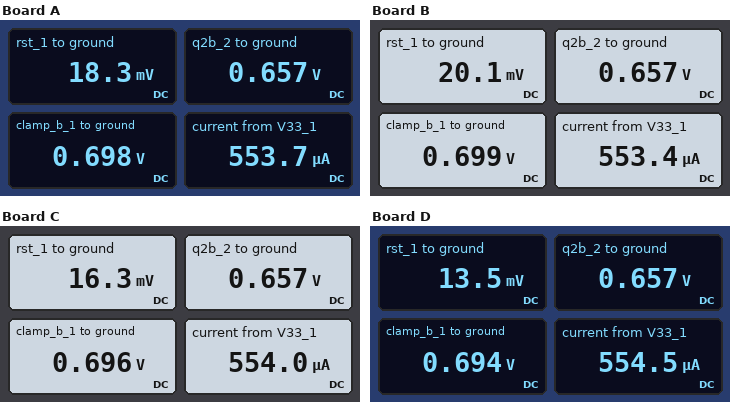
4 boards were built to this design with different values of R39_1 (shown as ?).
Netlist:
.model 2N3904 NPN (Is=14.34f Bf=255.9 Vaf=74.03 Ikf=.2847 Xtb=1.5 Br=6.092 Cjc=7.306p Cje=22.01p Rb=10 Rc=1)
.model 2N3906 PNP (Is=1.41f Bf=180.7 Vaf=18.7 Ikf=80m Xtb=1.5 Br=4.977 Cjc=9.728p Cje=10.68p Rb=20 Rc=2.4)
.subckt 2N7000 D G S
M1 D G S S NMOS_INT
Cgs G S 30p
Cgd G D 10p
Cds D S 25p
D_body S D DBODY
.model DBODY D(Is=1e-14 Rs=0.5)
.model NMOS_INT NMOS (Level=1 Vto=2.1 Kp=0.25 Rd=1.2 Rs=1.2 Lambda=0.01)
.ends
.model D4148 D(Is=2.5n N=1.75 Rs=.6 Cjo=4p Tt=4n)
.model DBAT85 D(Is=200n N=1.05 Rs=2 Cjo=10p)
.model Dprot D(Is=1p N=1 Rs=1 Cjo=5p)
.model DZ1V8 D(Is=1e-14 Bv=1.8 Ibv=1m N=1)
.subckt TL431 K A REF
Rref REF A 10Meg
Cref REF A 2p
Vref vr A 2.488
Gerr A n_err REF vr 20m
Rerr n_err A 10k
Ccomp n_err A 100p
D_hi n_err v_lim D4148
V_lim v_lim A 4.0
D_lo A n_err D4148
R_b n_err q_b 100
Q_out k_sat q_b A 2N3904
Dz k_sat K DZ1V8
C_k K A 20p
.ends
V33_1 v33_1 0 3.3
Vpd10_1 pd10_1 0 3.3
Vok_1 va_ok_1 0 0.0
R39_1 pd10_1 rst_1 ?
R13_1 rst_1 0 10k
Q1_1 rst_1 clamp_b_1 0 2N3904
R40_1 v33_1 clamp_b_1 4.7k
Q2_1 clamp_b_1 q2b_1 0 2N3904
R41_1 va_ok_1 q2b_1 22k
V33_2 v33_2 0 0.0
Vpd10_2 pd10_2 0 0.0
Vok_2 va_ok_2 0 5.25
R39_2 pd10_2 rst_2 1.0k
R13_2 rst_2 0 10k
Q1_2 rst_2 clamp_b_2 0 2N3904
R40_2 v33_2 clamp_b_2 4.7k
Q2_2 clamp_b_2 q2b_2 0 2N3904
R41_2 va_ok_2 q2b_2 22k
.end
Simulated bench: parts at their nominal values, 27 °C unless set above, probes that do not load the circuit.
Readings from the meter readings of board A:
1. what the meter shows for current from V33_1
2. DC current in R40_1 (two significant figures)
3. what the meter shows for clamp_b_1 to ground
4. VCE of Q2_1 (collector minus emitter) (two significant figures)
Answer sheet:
553.7 µA
550 µA
0.698 V
700 mV
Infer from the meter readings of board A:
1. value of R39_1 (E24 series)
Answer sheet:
1.5 kΩ
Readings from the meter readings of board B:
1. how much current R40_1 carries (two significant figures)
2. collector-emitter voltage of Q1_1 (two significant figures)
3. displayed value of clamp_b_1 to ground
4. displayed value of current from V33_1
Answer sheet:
550 µA
20 mV
0.699 V
553.4 µA
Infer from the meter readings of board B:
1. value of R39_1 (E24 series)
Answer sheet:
1.3 kΩ
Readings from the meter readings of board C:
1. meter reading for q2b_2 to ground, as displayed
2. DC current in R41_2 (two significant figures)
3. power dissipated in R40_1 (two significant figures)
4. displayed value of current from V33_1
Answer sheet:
0.657 V
210 µA
1.4 mW
554.0 µA
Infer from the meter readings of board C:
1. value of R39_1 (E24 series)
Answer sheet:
1.8 kΩ
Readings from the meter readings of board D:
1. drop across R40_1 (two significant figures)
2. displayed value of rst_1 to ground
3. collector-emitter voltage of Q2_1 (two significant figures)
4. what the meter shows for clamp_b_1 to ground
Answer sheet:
2.6 V
13.5 mV
690 mV
0.694 V
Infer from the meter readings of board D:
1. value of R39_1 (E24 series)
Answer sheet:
2.4 kΩ
